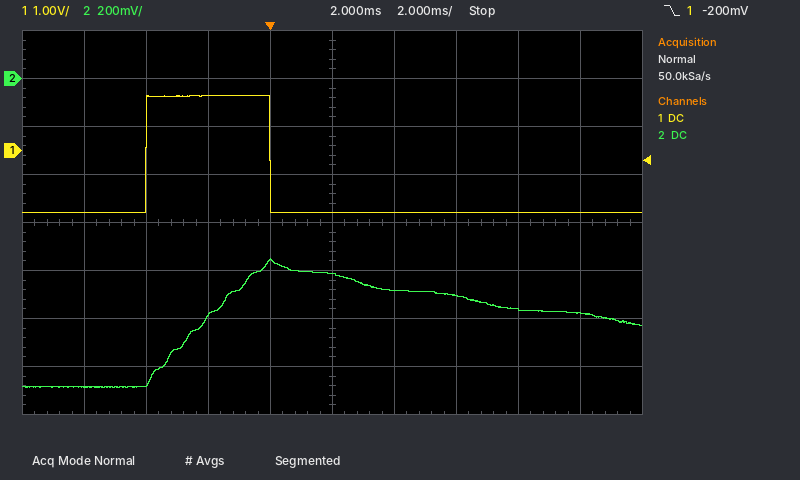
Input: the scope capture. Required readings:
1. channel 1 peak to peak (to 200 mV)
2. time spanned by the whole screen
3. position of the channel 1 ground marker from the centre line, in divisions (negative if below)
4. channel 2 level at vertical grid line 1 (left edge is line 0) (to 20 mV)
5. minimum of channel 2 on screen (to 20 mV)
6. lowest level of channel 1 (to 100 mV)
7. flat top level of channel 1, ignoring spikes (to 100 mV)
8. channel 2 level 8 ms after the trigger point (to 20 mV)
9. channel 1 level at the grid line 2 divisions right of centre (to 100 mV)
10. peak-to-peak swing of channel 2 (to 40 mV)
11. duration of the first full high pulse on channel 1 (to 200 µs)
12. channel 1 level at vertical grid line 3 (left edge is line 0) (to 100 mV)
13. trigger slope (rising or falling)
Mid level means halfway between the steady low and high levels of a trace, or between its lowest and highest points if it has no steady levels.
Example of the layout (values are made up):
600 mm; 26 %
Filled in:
2.4 V; 20 ms; +1.5 div; -1.28 V; -1.28 V; -1.3 V; 1.1 V; -960 mV; -1.3 V; 520 mV; 4.0 ms; 1.1 V; falling
